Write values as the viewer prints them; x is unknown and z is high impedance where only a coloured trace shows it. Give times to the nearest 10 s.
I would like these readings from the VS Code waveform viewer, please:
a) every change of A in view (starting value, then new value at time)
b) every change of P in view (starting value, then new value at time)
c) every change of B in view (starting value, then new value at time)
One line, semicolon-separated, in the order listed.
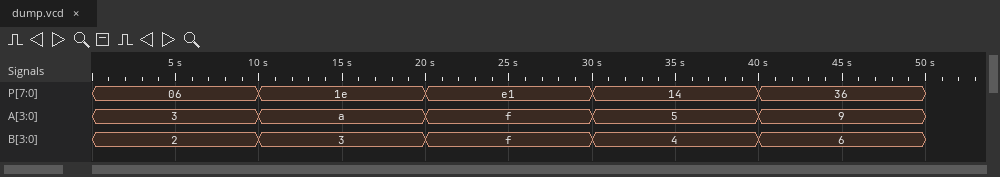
3, a at 10 s, f at 20 s, 5 at 30 s, 9 at 40 s; 06, 1e at 10 s, e1 at 20 s, 14 at 30 s, 36 at 40 s; 2, 3 at 10 s, f at 20 s, 4 at 30 s, 6 at 40 s
